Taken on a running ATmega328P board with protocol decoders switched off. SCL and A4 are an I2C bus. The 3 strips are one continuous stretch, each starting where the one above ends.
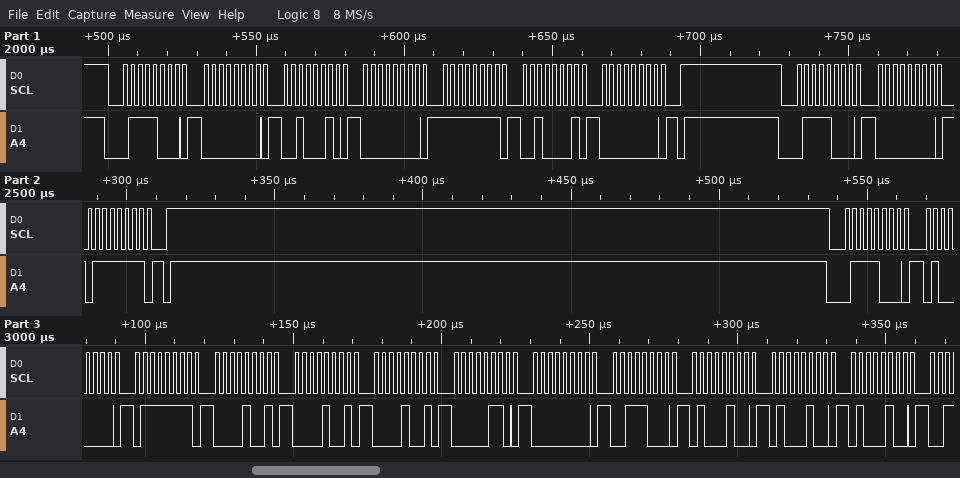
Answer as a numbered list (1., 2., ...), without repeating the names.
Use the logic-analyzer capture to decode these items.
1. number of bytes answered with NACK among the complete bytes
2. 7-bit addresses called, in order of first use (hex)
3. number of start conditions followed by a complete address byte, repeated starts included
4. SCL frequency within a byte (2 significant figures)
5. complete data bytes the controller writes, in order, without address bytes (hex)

1. 0
2. 0x3C
3. 3
4. 400 kHz
5. 00 22 00 FF 21 00 00 7F 40 7F 09 09 09 06 00 38 44 44 44
